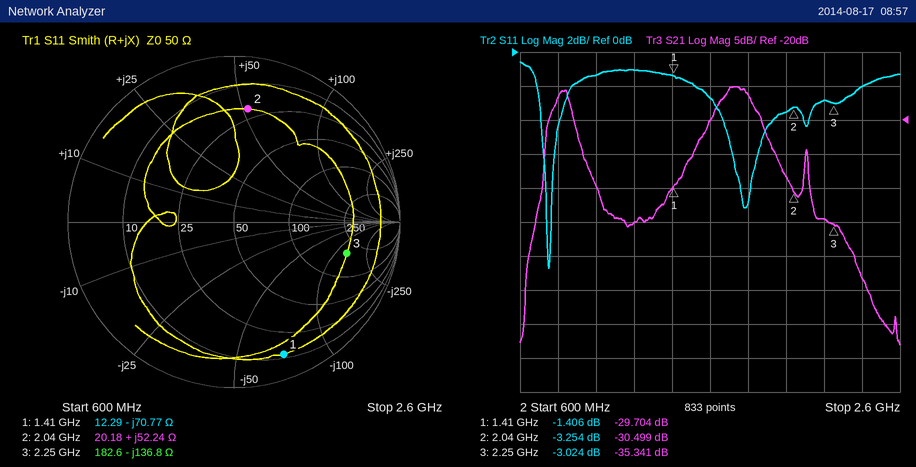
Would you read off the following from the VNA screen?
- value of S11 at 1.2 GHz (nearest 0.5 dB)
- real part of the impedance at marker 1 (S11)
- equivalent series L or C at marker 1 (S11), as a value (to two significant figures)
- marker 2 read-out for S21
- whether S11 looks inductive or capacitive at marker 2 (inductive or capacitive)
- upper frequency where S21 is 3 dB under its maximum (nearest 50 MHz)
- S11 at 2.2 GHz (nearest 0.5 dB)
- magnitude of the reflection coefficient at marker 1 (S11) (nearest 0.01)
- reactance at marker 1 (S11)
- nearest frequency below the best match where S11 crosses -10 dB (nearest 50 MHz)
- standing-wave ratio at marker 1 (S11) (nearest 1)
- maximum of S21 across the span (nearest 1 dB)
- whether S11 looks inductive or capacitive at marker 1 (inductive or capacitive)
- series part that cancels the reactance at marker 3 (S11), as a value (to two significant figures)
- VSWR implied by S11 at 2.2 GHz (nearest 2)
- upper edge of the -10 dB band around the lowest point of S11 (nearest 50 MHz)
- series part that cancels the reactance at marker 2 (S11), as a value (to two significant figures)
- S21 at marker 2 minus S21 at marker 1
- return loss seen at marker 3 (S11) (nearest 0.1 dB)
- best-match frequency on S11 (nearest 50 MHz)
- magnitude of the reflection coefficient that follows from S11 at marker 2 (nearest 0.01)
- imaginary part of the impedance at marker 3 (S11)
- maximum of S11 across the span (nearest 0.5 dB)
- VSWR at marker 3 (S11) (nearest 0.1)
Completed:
-1.0 dB
12.29 Ω
1.6 pF
-30.499 dB
inductive
1.85 GHz
-3.0 dB
0.85
-70.77 Ω
750 MHz
12
-15 dB
capacitive
9.7 nH
6
750 MHz
1.5 pF
-0.795 dB
3.0 dB
750 MHz
0.69
-136.8 Ω
-0.5 dB
5.8
